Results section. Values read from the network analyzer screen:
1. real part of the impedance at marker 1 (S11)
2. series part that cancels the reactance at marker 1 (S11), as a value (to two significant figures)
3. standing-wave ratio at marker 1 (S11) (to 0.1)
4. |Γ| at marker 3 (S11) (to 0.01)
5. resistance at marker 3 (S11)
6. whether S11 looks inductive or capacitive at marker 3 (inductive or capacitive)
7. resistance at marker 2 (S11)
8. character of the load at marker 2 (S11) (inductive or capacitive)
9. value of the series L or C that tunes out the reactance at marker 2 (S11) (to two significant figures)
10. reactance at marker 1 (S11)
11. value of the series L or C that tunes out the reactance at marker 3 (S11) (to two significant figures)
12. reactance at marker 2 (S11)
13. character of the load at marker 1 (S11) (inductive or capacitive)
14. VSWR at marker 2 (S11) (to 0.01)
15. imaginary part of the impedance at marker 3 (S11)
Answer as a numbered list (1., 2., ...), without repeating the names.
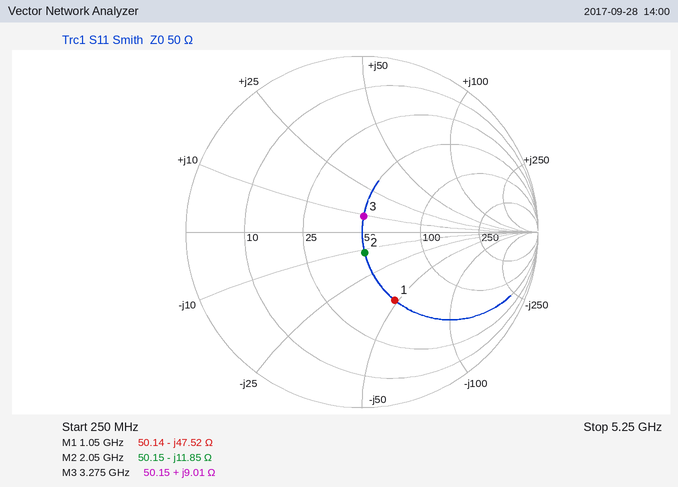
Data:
1. 50.14 Ω
2. 7.2 nH
3. 2.5
4. 0.09
5. 50.15 Ω
6. inductive
7. 50.15 Ω
8. capacitive
9. 920 pH
10. -47.52 Ω
11. 5.4 pF
12. -11.85 Ω
13. capacitive
14. 1.27
15. +9.01 Ω
